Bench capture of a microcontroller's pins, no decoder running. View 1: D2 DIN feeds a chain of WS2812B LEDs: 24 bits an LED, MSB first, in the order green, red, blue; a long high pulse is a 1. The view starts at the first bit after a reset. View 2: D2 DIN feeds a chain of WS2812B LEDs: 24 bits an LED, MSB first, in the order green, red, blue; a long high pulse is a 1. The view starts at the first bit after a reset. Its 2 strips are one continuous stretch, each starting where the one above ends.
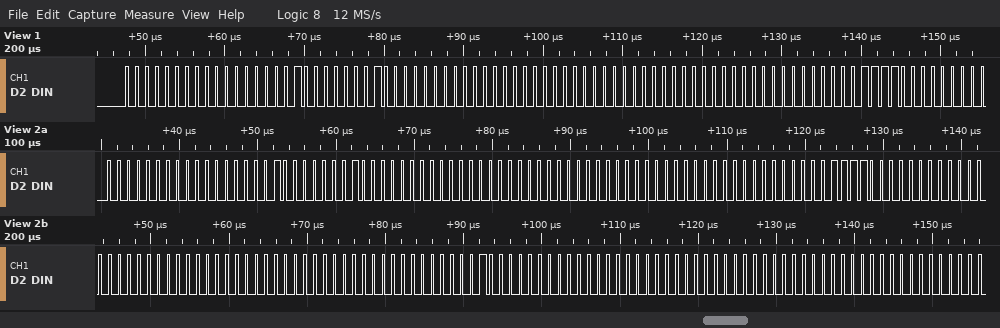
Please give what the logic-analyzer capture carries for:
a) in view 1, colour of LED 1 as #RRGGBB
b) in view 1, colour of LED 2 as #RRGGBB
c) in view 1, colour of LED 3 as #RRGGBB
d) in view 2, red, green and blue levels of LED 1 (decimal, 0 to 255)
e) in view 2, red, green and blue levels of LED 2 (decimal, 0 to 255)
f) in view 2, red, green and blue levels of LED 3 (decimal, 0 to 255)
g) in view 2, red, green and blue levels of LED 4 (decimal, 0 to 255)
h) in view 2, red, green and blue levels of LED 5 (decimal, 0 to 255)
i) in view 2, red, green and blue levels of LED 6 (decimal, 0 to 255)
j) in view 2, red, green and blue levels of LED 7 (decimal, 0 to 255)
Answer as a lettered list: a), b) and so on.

a) #000040
b) #004000
c) #000000
d) 0, 0, 64
e) 0, 64, 0
f) 0, 0, 0
g) 0, 60, 0
h) 0, 0, 0
i) 64, 0, 0
j) 0, 0, 0
